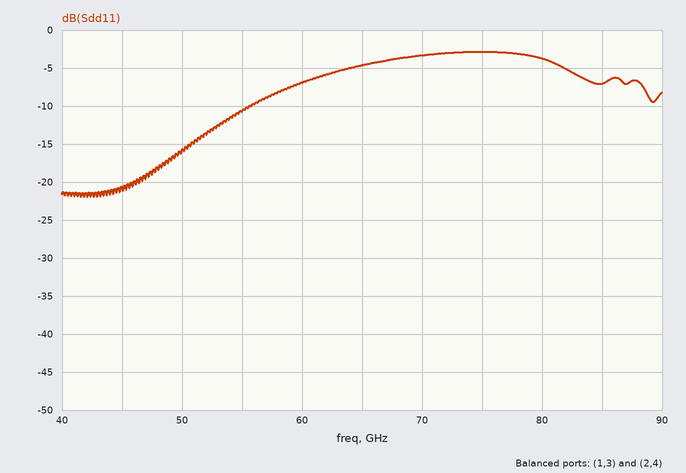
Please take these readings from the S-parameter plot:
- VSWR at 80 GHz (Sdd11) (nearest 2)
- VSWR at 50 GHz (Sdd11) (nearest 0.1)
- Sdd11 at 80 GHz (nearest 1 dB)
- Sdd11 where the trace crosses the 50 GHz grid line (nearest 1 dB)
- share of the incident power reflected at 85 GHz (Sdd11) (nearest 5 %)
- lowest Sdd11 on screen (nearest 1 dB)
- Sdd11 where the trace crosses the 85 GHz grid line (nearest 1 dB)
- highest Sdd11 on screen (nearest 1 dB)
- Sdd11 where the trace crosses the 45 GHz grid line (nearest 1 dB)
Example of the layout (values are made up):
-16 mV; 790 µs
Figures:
4; 1.4; -4 dB; -16 dB; 20 %; -22 dB; -7 dB; -3 dB; -21 dB
